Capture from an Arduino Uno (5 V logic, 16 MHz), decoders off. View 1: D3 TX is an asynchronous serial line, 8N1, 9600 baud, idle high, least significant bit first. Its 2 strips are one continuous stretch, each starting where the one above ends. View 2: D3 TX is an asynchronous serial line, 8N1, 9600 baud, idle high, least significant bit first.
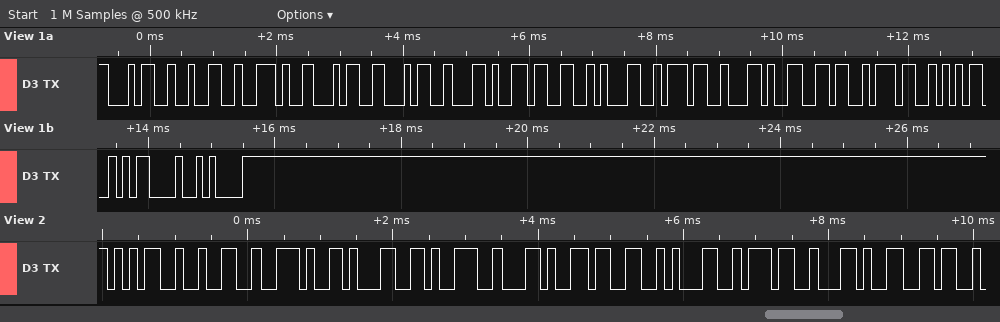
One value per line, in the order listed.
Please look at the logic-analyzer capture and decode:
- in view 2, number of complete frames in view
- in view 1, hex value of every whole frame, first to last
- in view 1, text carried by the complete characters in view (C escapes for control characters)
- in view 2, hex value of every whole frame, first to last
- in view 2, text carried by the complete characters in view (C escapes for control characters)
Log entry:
11
0x34 0x32 0x2E 0x34 0x34 0x2C 0x33 0x31 0x37 0x2C 0x36 0x37 0x35 0x0D 0x0A
"42.44,317,675\r\n"
35 32 2E 31 39 2C 33 31 37 2C 36
"52.19,317,6"
